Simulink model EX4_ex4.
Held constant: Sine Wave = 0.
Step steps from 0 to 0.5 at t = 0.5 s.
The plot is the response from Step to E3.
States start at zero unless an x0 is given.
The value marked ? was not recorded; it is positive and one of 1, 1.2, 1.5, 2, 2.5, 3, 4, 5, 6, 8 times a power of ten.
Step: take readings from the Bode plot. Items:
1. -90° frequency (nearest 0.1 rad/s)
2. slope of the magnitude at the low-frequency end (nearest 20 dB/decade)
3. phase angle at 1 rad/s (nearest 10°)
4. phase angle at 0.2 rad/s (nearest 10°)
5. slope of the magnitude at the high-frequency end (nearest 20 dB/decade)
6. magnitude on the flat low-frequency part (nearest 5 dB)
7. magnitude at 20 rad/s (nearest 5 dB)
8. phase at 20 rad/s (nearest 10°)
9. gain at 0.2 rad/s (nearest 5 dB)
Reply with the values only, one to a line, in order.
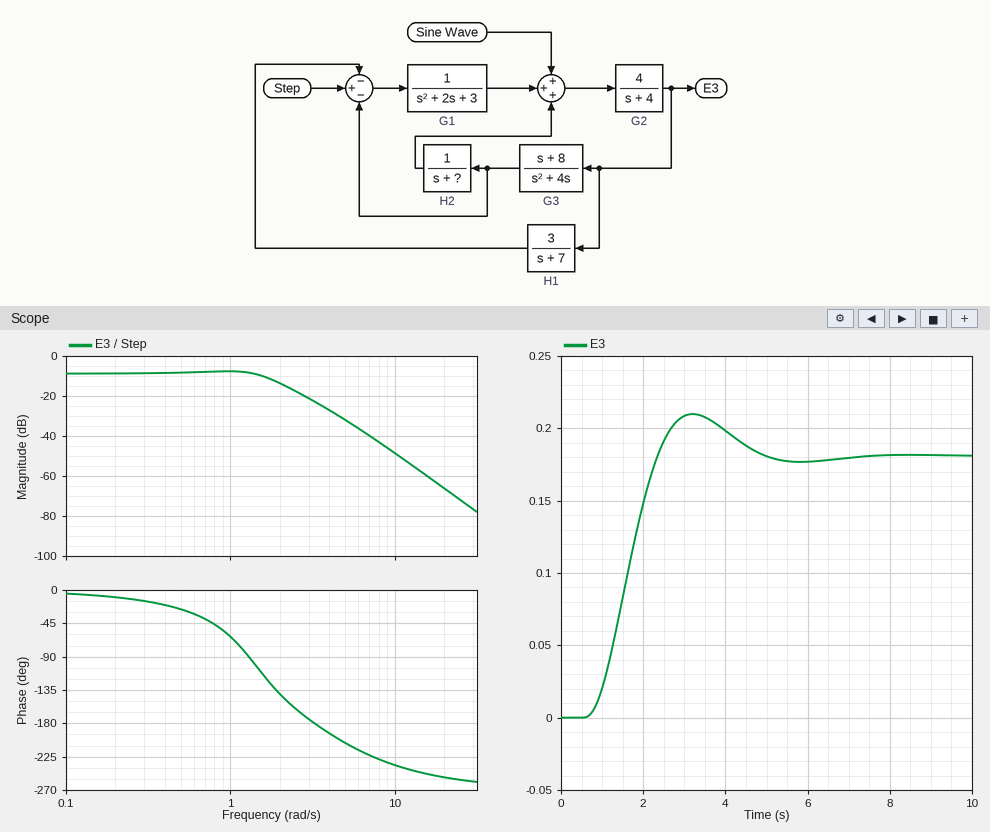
1.3 rad/s
0 dB/decade
-60°
-10°
-60 dB/decade
-10 dB
-65 dB
-250°
-10 dB
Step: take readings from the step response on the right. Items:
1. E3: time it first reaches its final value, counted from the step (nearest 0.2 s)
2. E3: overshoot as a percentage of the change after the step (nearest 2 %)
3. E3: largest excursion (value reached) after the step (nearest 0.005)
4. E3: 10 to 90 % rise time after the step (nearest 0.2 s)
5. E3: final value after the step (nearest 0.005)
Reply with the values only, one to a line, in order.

1.8 s
16 %
0.210
1.2 s
0.180
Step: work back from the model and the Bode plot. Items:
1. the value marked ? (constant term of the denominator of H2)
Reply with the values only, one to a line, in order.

3
